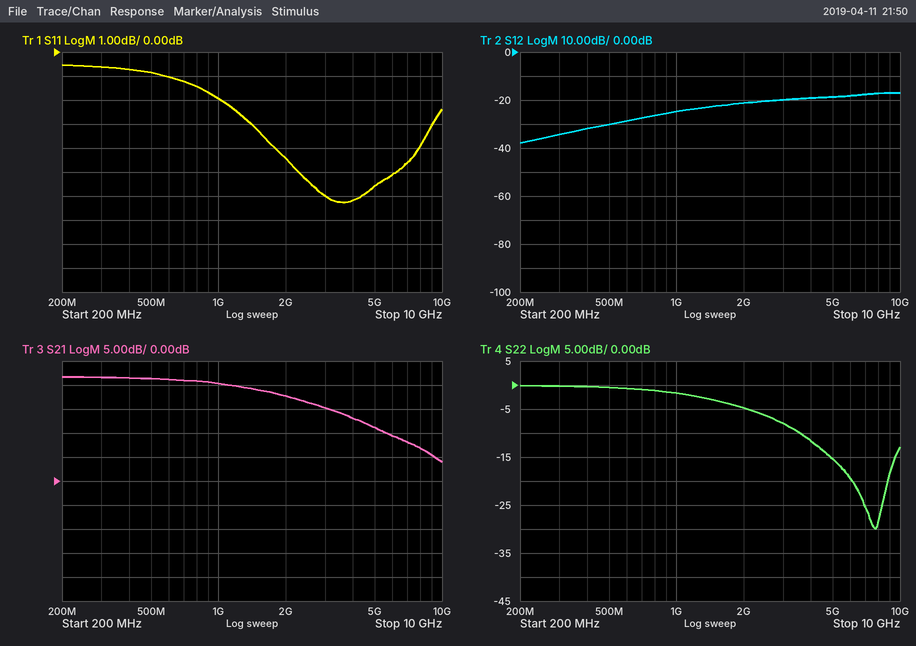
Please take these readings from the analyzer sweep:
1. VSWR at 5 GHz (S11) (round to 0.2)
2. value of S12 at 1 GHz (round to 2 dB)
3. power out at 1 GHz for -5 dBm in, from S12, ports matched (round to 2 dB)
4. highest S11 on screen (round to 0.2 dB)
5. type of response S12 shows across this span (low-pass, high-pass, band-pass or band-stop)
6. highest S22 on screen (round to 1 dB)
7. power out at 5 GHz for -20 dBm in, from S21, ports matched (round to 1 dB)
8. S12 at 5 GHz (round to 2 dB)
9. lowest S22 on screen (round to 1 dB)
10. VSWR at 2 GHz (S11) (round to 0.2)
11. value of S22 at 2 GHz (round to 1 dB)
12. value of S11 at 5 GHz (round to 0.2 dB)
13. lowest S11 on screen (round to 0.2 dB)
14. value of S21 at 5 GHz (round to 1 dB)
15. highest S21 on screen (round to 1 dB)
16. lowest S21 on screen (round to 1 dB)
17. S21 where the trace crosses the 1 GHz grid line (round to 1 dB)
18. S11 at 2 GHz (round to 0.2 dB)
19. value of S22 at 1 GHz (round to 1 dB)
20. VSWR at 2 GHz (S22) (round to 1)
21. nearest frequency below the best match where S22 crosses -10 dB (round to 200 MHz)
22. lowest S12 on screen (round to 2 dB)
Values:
3.2
-24 dB
-30 dBm
-0.6 dB
high-pass
0 dB
-9 dBm
-18 dB
-30 dB
4.0
-5 dB
-5.6 dB
-6.2 dB
11 dB
22 dB
4 dB
20 dB
-4.4 dB
-2 dB
4
3.6 GHz
-38 dB
